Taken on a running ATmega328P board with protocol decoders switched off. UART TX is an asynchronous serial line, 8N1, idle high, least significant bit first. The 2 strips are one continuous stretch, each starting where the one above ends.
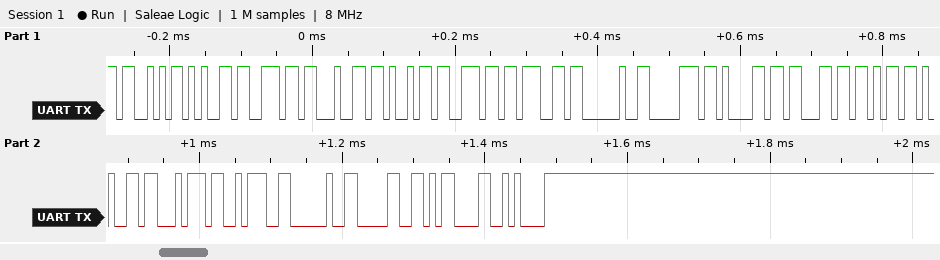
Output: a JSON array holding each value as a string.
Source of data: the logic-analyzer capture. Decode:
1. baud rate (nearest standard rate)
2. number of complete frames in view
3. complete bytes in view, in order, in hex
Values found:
["115200 baud", "19", "0x53 0x65 0x6E 0x64 0x69 0x6E 0x67 0x20 0x70 0x61 0x63 0x6B 0x65 0x74 0x3A 0x20 0x30 0x0D 0x0A"]
